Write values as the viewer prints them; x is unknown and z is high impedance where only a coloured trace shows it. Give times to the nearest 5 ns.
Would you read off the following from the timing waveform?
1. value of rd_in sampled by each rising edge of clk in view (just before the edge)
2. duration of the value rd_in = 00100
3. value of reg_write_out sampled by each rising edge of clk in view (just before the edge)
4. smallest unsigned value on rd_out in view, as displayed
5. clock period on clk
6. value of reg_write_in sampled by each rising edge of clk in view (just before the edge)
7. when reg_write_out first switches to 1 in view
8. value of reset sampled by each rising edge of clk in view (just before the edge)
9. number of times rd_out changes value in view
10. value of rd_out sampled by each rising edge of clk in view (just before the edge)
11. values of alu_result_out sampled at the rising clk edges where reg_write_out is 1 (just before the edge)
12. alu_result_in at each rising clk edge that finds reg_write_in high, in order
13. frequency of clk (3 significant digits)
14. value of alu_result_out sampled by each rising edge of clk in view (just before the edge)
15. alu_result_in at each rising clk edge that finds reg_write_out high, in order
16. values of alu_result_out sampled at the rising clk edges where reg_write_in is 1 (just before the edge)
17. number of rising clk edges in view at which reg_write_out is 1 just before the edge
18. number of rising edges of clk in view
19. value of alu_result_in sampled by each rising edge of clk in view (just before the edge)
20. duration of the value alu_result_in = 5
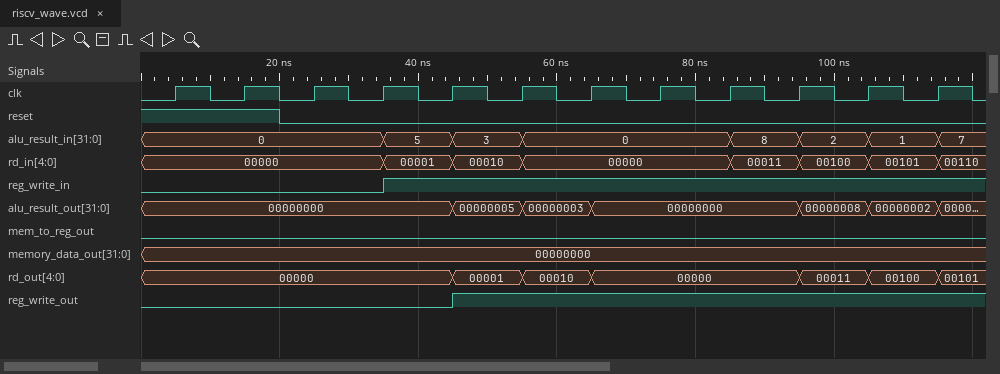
00000, 00000, 00000, 00000, 00001, 00010, 00000, 00000, 00000, 00011, 00100, 00101
10 ns
0 0 0 0 0 1 1 1 1 1 1 1
00000
10 ns
0 0 0 0 1 1 1 1 1 1 1 1
45 ns
1 1 0 0 0 0 0 0 0 0 0 0
6
00000, 00000, 00000, 00000, 00000, 00001, 00010, 00000, 00000, 00000, 00011, 00100
00000005, 00000003, 00000000, 00000000, 00000000, 00000008, 00000002
5, 3, 0, 0, 0, 8, 2, 1
100 MHz
00000000, 00000000, 00000000, 00000000, 00000000, 00000005, 00000003, 00000000, 00000000, 00000000, 00000008, 00000002
3, 0, 0, 0, 8, 2, 1
00000000, 00000005, 00000003, 00000000, 00000000, 00000000, 00000008, 00000002
7
12
0, 0, 0, 0, 5, 3, 0, 0, 0, 8, 2, 1
10 ns
